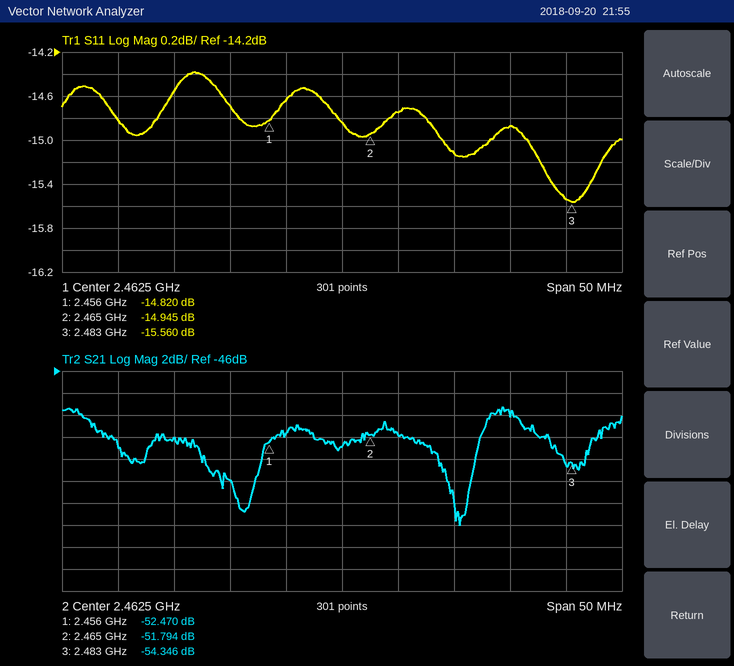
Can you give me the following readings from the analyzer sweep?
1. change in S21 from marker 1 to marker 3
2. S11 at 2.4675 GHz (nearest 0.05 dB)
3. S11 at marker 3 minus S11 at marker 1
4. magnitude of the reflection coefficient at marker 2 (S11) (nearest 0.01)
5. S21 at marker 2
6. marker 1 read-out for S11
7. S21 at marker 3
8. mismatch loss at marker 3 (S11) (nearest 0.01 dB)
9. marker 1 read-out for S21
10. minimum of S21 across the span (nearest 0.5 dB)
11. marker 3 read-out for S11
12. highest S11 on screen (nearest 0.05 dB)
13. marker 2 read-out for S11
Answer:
-1.876 dB
-14.75 dB
-0.740 dB
0.18
-51.794 dB
-14.820 dB
-54.346 dB
0.12 dB
-52.470 dB
-60.0 dB
-15.560 dB
-14.40 dB
-14.945 dB
